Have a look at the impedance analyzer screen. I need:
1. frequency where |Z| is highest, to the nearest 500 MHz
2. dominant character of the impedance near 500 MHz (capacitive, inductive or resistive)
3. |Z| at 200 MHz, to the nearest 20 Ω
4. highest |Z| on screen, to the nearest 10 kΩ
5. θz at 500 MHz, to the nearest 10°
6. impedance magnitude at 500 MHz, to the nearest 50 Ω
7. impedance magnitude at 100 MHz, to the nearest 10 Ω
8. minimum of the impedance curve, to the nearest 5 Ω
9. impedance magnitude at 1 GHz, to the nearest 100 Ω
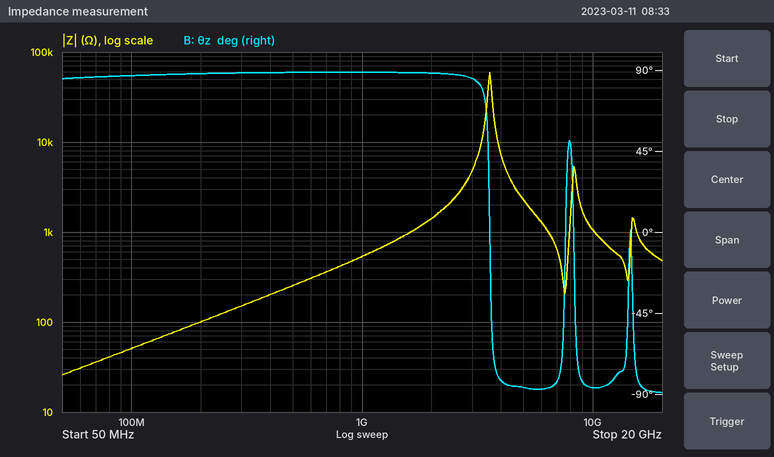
3.5 GHz
inductive
100 Ω
60 kΩ
90°
250 Ω
50 Ω
25 Ω
500 Ω
